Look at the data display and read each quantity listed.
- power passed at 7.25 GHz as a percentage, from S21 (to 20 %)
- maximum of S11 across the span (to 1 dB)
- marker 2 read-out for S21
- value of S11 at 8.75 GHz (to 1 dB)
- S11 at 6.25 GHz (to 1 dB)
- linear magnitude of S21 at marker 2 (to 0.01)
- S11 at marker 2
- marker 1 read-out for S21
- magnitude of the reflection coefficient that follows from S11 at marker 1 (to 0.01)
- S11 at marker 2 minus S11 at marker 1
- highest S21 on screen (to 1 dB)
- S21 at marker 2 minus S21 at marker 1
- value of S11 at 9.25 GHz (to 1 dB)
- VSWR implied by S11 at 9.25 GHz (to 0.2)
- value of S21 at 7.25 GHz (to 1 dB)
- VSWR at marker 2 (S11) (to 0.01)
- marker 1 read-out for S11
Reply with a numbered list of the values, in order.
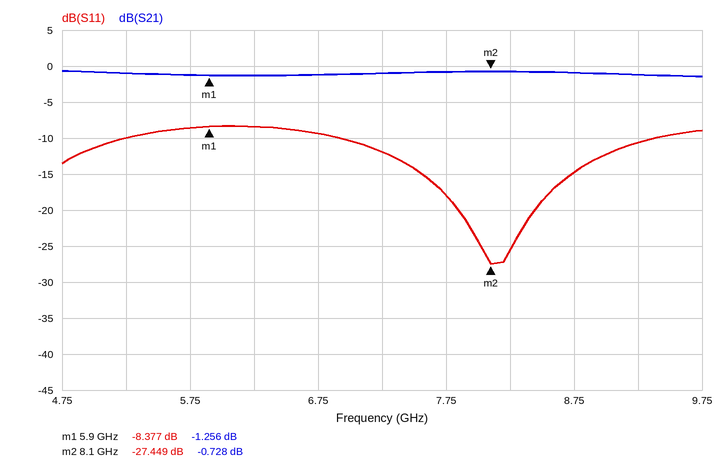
1. 80 %
2. -8 dB
3. -0.728 dB
4. -15 dB
5. -8 dB
6. 0.92
7. -27.449 dB
8. -1.256 dB
9. 0.38
10. -19.072 dB
11. -1 dB
12. 0.528 dB
13. -11 dB
14. 1.8
15. -1 dB
16. 1.09
17. -8.377 dB
